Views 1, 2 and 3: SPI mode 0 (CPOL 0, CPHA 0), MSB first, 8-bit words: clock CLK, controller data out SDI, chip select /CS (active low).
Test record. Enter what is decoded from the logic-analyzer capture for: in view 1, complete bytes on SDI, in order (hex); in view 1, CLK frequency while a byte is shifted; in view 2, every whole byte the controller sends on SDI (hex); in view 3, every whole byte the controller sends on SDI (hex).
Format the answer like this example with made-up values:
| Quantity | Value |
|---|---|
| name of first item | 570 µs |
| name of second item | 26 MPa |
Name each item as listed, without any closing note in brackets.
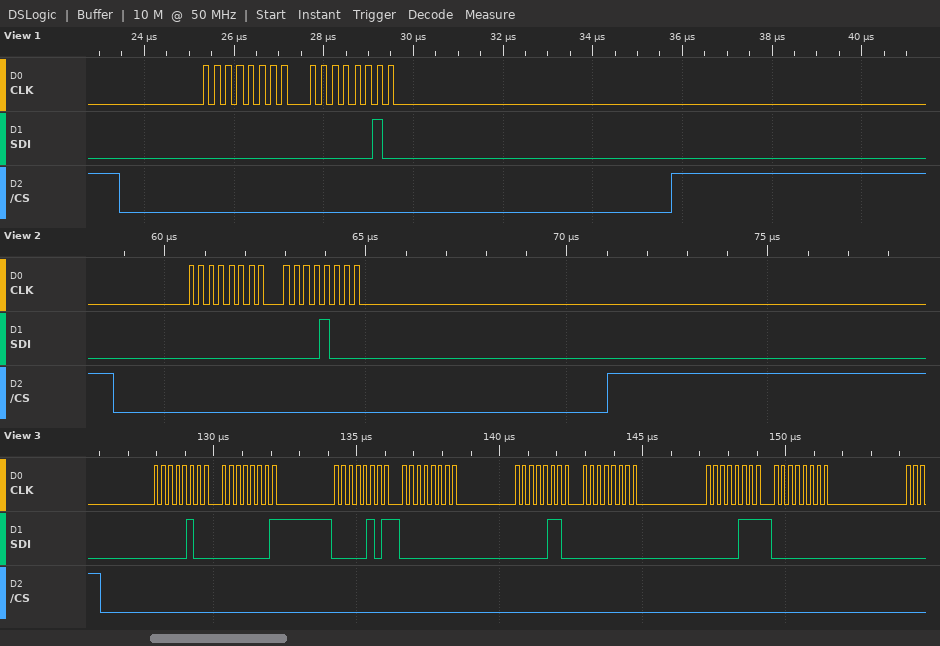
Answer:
| Quantity | Value |
|---|---|
| in view 1, complete bytes on SDI, in order | 0x00 0x02 |
| in view 1, CLK frequency while a byte is shifted | 4 MHz |
| in view 2, every whole byte the controller sends on SDI | 00 08 |
| in view 3, every whole byte the controller sends on SDI | 04 01 05 00 06 00 07 00 |
